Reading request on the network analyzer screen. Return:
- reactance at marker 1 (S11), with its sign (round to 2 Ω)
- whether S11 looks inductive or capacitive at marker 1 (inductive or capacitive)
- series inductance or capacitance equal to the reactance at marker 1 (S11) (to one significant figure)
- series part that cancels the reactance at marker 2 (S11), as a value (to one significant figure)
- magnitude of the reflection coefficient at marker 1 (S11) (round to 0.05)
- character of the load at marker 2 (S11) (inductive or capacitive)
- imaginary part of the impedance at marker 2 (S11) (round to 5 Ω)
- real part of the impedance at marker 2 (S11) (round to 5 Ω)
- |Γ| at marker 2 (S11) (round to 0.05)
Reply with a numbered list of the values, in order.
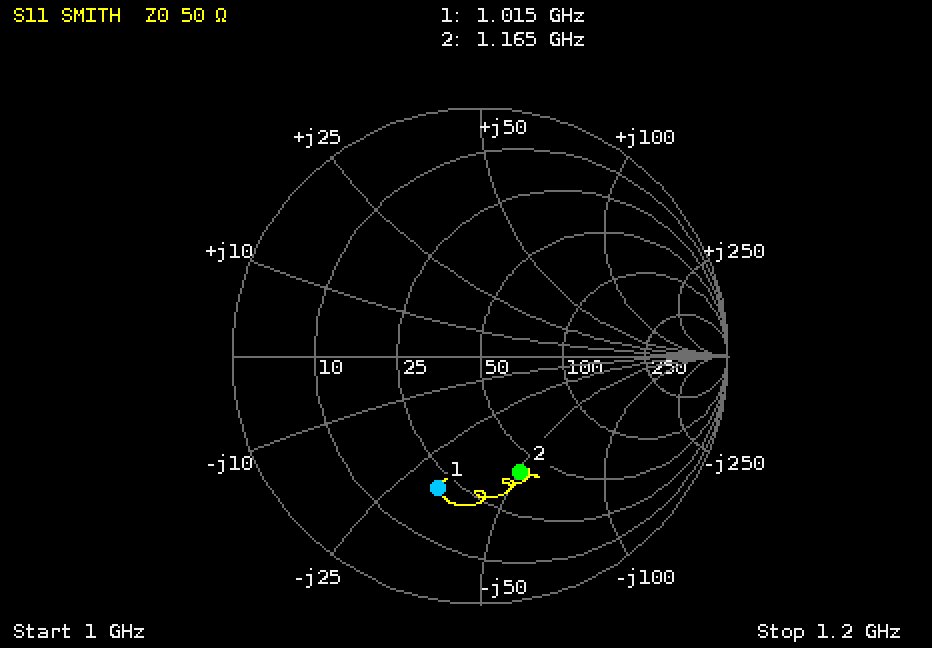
1. -32 Ω
2. capacitive
3. 5 pF
4. 7 nH
5. 0.55
6. capacitive
7. -50 Ω
8. 40 Ω
9. 0.50
